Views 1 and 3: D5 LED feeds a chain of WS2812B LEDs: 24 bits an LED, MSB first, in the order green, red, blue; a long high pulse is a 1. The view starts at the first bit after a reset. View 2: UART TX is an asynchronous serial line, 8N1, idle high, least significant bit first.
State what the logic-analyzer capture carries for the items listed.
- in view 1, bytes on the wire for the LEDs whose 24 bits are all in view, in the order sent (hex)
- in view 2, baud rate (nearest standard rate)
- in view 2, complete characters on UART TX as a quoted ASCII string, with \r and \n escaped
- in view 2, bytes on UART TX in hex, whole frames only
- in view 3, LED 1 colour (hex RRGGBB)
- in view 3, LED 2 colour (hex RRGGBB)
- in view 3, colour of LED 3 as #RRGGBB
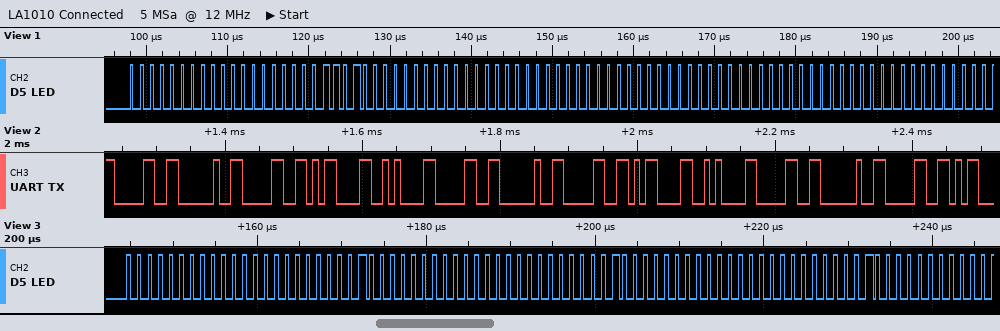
00 00 1A 00 00 00 00 00 00
115200 baud
"0 0\r\n0 0\r\n0 0"
30 20 30 0D 0A 30 20 30 0D 0A 30 20 30
#000002
#000002
#000002
